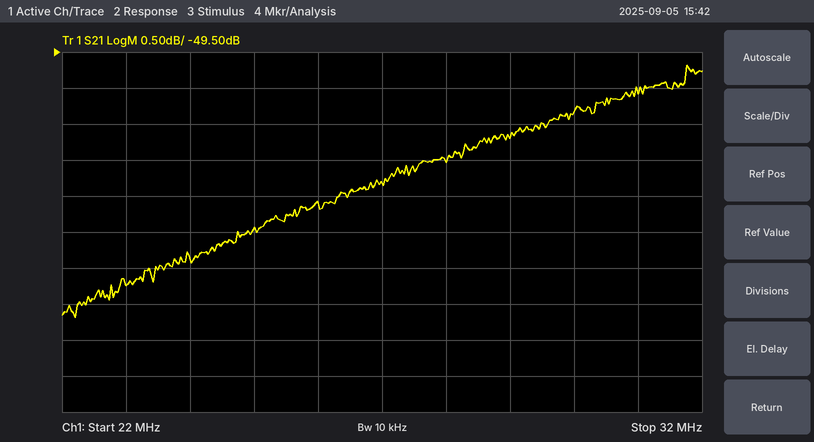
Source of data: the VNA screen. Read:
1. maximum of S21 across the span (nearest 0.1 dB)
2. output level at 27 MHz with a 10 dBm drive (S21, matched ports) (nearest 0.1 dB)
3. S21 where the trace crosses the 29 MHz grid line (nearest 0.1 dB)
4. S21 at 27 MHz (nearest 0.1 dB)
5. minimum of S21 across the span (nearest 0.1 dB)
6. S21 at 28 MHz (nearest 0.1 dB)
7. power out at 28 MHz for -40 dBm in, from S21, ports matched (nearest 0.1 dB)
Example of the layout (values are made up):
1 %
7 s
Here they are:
-49.7 dB
-41.3 dBm
-50.7 dB
-51.3 dB
-53.2 dB
-51.0 dB
-91.0 dBm
